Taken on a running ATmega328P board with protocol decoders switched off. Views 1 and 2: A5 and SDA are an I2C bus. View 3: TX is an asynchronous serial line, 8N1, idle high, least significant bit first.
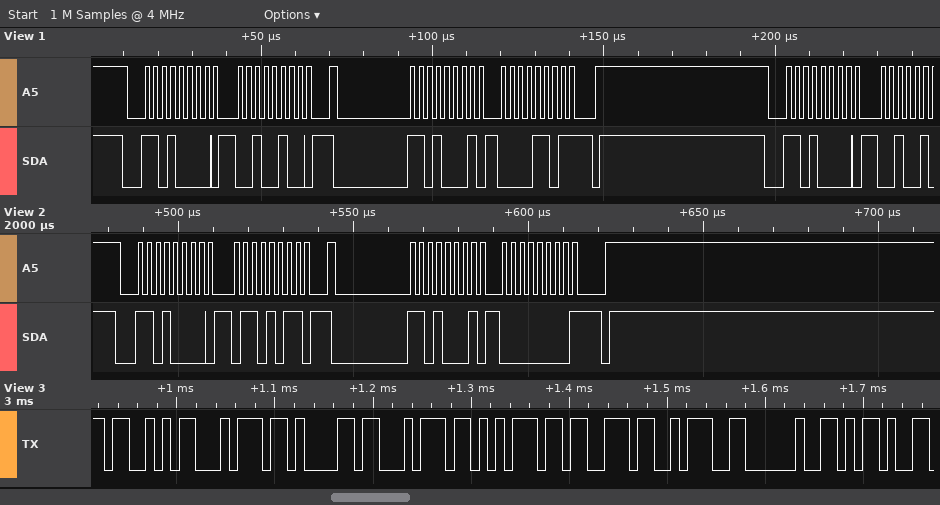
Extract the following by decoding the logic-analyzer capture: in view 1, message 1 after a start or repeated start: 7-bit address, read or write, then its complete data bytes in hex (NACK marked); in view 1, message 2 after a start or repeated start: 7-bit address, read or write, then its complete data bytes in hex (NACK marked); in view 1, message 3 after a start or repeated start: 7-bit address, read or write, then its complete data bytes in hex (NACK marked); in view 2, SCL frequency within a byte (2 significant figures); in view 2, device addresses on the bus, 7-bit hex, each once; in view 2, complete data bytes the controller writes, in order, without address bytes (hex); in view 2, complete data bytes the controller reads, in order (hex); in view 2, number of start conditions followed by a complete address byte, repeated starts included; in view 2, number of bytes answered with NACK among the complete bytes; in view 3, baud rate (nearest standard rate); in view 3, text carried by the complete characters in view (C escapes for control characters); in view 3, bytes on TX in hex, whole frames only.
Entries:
0x68 write: 24
0x68 read: 0D NACK
0x68 write
400 kHz
0x68
6B
00
2
1
115200 baud
"Status: -"
53 74 61 74 75 73 3A 20 2D
